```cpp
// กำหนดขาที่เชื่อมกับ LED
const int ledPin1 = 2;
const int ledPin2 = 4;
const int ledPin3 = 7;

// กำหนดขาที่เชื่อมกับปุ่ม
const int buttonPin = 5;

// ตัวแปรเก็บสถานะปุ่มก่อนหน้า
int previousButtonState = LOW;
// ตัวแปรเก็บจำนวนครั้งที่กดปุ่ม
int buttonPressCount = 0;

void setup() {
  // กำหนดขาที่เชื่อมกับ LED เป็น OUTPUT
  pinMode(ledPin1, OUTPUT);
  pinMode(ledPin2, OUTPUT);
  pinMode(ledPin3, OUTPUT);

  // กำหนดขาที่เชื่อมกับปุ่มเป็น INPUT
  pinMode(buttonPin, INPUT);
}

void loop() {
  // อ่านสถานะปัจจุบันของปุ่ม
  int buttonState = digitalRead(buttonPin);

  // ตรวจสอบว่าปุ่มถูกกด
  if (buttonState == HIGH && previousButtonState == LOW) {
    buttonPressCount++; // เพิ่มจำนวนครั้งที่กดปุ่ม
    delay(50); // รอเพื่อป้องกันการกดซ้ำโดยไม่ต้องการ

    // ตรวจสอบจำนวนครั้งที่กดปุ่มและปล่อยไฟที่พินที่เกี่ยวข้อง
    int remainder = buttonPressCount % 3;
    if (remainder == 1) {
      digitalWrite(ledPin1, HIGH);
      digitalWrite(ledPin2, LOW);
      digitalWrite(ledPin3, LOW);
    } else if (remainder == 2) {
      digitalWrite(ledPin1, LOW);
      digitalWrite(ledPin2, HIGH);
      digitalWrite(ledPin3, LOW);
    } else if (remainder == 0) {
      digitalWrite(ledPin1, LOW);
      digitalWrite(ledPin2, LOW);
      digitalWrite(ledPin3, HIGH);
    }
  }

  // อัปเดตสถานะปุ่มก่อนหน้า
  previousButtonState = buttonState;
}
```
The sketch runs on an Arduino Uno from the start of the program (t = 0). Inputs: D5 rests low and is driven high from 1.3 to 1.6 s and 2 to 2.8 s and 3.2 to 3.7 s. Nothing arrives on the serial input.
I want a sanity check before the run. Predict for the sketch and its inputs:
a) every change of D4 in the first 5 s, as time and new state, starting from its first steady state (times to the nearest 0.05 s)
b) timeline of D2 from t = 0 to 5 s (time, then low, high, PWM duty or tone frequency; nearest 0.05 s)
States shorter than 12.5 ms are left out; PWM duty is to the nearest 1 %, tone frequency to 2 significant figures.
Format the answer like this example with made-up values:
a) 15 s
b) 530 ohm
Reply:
a) 0 s low; 2.05 s high; 3.25 s low
b) 0 s low; 1.35 s high; 2.05 s low
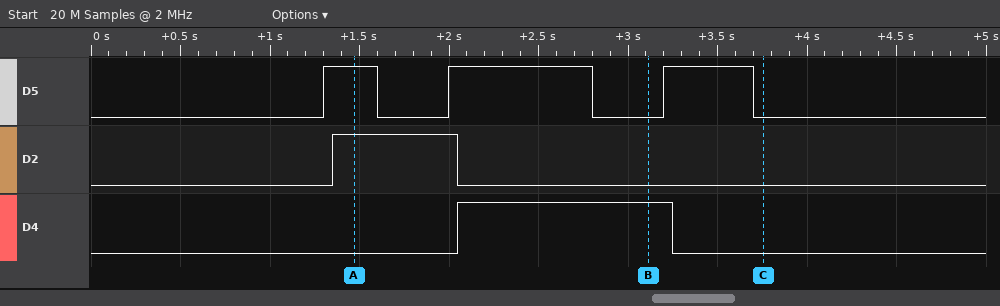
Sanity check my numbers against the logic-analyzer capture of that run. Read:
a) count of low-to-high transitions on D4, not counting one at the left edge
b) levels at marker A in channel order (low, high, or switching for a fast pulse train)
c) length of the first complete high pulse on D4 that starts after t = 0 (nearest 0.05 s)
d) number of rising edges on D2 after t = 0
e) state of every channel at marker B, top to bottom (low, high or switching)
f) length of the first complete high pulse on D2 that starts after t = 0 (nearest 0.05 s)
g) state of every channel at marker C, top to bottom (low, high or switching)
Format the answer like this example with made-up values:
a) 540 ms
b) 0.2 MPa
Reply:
a) 1
b) D5 high, D2 high, D4 low
c) 1.20 s
d) 1
e) D5 low, D2 low, D4 high
f) 0.70 s
g) D5 low, D2 low, D4 low
